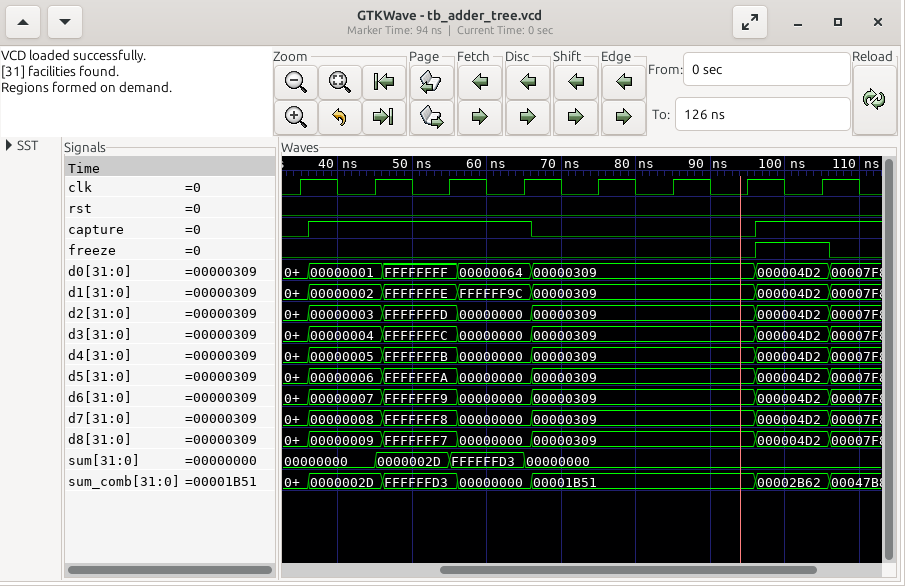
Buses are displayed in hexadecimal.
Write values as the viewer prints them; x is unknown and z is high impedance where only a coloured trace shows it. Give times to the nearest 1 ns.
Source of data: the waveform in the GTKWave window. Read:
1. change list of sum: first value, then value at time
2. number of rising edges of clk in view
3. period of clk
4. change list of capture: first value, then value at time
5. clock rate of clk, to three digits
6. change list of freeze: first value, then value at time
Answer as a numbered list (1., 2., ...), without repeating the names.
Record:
1. 00000000, 0000002D at 45 ns, FFFFFFD3 at 55 ns, 00000000 at 65 ns
2. 8
3. 10 ns
4. 0, 1 at 36 ns, 0 at 66 ns, 1 at 96 ns
5. 100 MHz
6. 0, 1 at 96 ns, 0 at 106 ns
